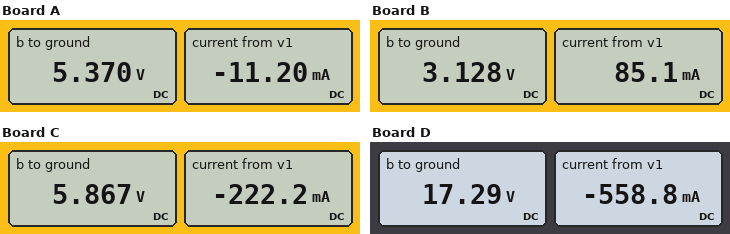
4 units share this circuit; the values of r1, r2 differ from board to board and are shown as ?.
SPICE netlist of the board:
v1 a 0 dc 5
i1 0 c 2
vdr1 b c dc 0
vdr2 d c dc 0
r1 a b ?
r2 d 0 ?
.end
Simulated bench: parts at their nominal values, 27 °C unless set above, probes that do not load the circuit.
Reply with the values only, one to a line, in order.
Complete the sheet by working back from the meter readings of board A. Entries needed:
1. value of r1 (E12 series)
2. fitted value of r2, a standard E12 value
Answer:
33 Ω
2.7 Ω
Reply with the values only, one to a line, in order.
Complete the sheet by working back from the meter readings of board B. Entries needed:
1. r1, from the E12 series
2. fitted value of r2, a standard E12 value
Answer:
22 Ω
1.5 Ω
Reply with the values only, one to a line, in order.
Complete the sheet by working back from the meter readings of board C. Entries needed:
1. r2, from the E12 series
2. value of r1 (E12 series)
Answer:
3.3 Ω
3.9 Ω
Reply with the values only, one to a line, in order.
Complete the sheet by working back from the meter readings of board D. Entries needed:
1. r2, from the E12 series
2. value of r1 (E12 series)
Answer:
12 Ω
22 Ω
